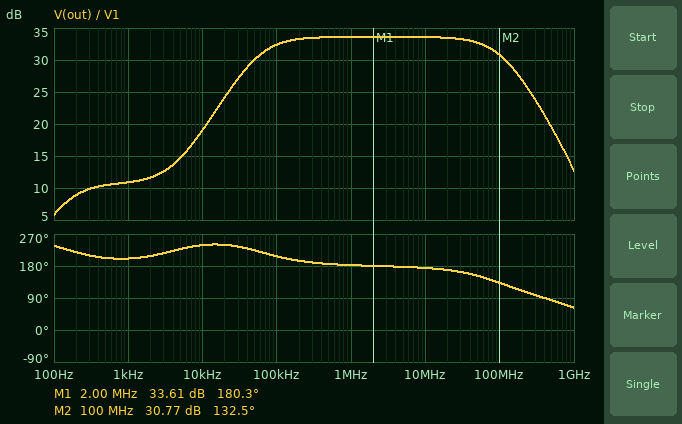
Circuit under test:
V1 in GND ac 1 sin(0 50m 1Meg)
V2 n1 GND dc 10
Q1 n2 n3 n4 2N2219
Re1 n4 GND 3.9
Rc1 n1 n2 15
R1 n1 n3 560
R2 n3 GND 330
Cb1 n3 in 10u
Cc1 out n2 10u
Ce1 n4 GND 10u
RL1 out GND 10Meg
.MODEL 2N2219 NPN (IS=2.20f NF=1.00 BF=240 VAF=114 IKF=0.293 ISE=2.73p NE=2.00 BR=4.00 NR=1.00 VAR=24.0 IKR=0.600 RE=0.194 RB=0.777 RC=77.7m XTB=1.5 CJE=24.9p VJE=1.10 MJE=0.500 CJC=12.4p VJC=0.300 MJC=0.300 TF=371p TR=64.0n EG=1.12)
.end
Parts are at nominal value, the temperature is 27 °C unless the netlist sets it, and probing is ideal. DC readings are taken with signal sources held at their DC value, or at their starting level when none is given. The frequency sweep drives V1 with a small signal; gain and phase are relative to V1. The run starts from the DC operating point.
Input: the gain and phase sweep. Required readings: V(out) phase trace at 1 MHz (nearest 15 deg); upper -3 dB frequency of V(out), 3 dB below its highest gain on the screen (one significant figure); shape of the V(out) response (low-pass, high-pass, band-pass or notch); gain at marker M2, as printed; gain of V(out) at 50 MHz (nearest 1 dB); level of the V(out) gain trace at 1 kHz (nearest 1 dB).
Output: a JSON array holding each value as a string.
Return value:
["180 deg", "100 MHz", "band-pass", "30.77 dB", "33 dB", "11 dB"]
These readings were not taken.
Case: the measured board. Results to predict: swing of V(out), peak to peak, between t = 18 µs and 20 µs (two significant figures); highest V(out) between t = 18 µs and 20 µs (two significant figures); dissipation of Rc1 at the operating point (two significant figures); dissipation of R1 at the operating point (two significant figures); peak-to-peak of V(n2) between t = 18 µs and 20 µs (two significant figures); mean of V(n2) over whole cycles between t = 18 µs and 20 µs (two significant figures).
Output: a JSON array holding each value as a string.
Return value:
["3.7 V", "2.3 V", "2.9 W", "95 mW", "3.7 V", "3.5 V"]
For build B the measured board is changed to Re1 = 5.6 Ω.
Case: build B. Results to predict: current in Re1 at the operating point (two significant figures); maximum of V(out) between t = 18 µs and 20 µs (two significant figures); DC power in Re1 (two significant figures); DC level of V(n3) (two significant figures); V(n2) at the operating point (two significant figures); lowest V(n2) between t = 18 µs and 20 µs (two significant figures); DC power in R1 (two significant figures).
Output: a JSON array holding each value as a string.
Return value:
["360 mA", "2.2 V", "740 mW", "3.0 V", "4.6 V", "2.4 V", "88 mW"]
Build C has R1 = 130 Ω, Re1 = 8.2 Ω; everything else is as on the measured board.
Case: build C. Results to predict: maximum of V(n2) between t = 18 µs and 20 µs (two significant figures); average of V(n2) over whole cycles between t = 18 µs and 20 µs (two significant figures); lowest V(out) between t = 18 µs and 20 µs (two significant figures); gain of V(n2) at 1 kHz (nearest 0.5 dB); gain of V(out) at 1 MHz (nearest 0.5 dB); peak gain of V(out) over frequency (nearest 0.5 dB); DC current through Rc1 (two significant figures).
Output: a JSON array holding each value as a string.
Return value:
["4.2 V", "3.8 V", "-16 mV", "-12.5 dB", "-8.5 dB", "-5.5 dB", "410 mA"]
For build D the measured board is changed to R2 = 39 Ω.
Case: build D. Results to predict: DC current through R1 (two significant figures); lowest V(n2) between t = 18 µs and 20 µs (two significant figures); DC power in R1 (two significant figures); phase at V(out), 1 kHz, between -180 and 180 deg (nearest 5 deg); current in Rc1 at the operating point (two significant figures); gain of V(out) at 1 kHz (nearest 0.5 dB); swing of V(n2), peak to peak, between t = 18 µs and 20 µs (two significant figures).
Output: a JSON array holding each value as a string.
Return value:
["17 mA", "10 V", "160 mW", "-155 deg", "190 µA", "-20.0 dB", "19 mV"]
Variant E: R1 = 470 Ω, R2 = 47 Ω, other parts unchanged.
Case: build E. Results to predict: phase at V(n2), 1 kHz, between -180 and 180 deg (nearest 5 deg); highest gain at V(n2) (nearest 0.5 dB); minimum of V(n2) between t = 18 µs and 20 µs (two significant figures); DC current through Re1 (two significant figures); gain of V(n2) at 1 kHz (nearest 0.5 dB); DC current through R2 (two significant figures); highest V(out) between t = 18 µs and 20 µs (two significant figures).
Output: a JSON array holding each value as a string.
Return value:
["-150 deg", "22.0 dB", "8.8 V", "29 mA", "9.0 dB", "19 mA", "380 mV"]
